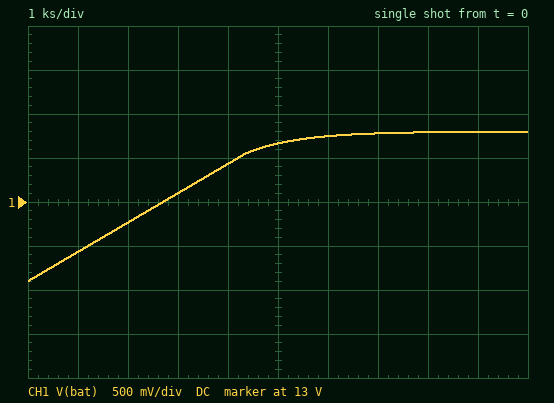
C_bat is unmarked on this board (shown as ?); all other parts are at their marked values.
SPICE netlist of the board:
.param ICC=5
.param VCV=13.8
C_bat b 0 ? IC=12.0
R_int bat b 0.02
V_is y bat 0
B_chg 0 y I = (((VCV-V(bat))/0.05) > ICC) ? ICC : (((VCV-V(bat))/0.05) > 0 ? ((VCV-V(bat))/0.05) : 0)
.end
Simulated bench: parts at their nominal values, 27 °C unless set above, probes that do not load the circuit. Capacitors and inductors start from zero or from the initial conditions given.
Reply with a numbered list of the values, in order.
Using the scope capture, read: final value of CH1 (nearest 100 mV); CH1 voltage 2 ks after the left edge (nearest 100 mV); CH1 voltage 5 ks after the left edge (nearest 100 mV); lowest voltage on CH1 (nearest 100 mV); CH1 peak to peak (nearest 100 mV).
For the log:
1. 13.8 V
2. 12.8 V
3. 13.7 V
4. 12.1 V
5. 1.7 V
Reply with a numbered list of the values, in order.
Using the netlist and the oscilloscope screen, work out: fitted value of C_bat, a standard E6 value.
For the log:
1. 15 kF
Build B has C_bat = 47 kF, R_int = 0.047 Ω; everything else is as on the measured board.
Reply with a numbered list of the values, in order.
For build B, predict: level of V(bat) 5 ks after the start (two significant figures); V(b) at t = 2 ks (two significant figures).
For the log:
1. 13 V
2. 12 V
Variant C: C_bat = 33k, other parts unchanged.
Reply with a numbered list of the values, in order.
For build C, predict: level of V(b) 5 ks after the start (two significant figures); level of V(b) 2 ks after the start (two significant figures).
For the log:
1. 13 V
2. 12 V
